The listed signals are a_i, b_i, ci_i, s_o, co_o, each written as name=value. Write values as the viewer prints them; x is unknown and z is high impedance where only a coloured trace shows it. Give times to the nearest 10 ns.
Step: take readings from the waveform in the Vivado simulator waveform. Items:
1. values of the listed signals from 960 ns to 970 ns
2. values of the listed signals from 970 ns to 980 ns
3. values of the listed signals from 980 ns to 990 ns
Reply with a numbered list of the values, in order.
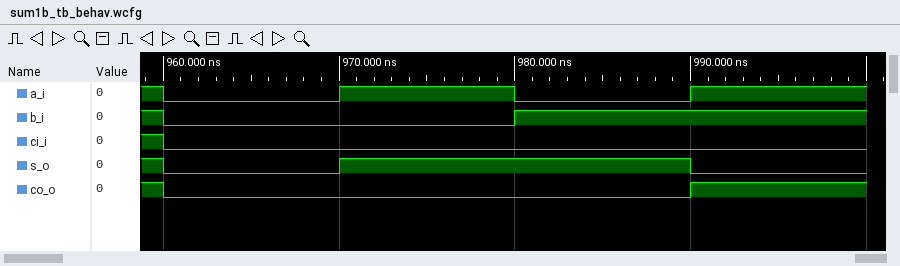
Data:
1. a_i=0, b_i=0, ci_i=0, s_o=0, co_o=0
2. a_i=1, b_i=0, ci_i=0, s_o=1, co_o=0
3. a_i=0, b_i=1, ci_i=0, s_o=1, co_o=0
